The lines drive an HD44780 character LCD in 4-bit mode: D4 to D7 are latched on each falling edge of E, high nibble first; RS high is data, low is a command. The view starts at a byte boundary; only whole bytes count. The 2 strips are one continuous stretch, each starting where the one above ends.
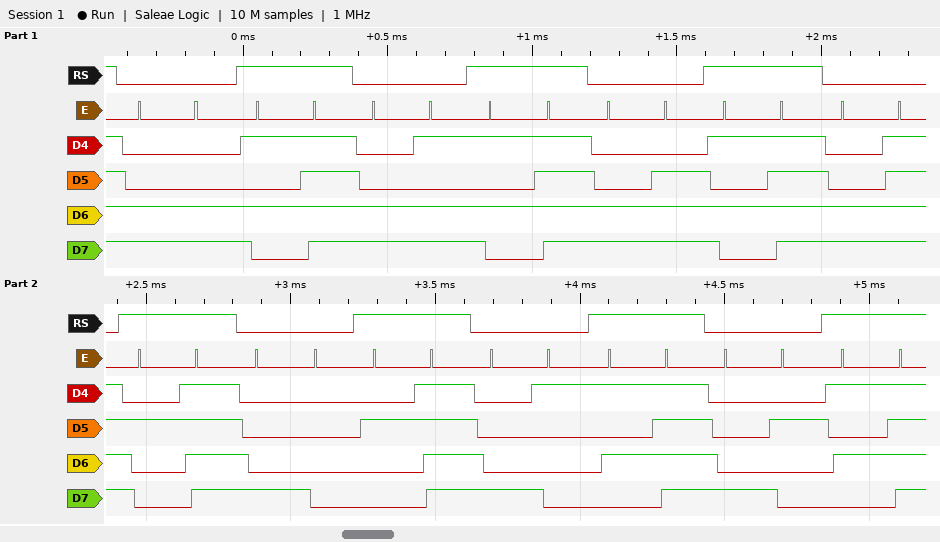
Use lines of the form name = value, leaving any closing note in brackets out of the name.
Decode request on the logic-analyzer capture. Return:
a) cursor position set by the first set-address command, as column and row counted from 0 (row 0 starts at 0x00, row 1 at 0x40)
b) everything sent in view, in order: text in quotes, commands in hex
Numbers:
cursor position set by the first set-address command, as column and row counted from 0 = column 12, row 1
everything sent in view, in order: text in quotes, commands in hex = 0xCC "_" 0xCD "_" 0xCE "_" 0xCF "/" 0x80 "/" 0x81 "_" 0x82 "_"
